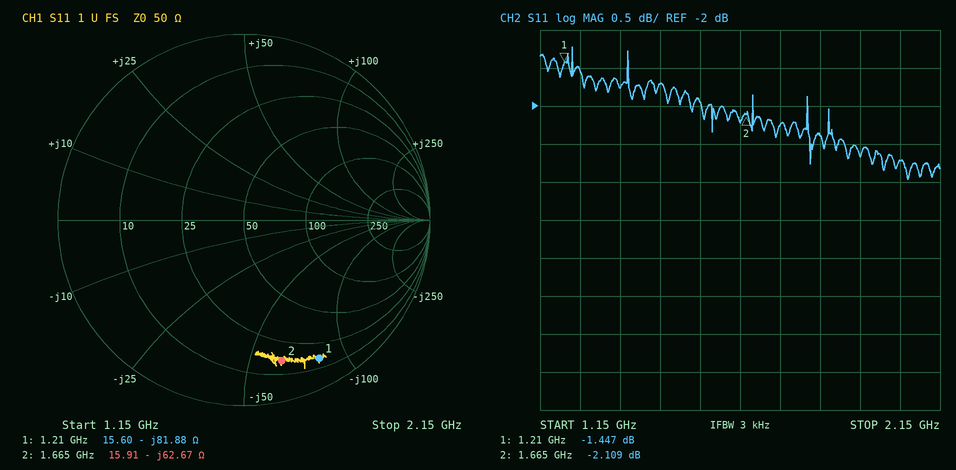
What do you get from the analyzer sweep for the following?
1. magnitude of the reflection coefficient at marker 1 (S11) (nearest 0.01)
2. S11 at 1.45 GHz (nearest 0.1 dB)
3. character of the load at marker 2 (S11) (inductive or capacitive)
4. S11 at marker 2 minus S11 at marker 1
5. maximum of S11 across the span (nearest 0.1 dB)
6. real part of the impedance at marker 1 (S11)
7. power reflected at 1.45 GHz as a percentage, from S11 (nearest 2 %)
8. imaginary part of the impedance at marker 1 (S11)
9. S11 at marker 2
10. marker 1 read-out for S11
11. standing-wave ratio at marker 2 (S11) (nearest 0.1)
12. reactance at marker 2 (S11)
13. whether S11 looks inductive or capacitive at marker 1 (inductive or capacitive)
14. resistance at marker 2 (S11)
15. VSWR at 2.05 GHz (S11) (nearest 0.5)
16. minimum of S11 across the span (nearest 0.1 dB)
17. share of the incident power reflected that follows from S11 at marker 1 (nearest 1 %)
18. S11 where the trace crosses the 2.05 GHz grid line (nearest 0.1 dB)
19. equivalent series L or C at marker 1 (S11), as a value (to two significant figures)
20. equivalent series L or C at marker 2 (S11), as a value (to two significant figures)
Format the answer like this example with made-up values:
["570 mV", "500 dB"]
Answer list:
["0.85", "-1.7 dB", "capacitive", "-0.662 dB", "-1.2 dB", "15.60 Ω", "68 %", "-81.88 Ω", "-2.109 dB", "-1.447 dB", "8.3", "-62.67 Ω", "capacitive", "15.91 Ω", "6.5", "-3.0 dB", "72 %", "-2.7 dB", "1.6 pF", "1.5 pF"]
